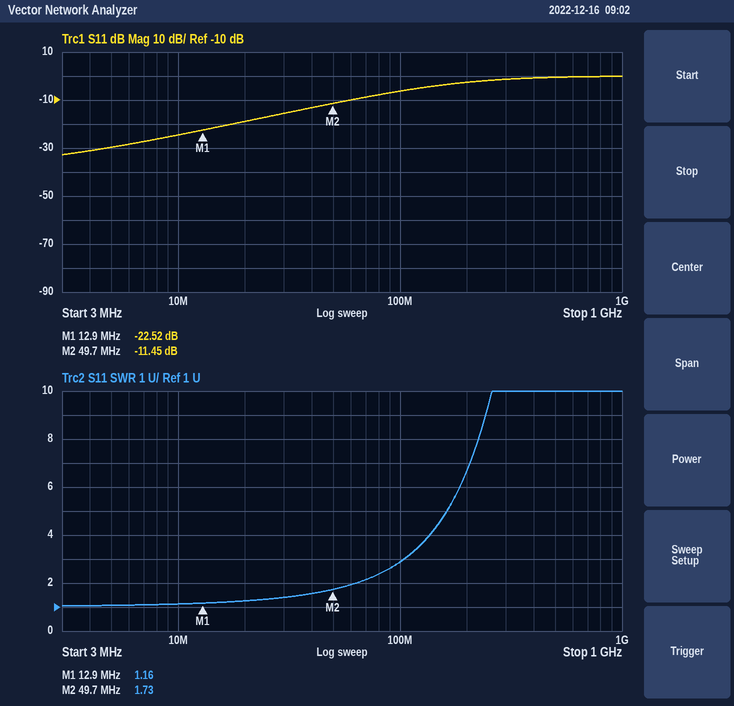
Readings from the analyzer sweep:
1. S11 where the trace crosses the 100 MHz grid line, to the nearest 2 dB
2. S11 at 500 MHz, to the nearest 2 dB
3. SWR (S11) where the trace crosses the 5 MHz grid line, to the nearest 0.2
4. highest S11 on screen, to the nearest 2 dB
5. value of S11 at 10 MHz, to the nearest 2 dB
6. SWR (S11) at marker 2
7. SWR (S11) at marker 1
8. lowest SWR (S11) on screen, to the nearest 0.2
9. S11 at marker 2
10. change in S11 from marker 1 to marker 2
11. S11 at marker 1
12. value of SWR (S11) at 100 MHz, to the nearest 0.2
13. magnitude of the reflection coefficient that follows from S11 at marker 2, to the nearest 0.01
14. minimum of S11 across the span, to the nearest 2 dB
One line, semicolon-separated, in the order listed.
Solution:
-6 dB; 0 dB; 1.0; 0 dB; -24 dB; 1.73; 1.16; 1.0; -11.45 dB; 11.07 dB; -22.52 dB; 2.8; 0.27; -32 dB
